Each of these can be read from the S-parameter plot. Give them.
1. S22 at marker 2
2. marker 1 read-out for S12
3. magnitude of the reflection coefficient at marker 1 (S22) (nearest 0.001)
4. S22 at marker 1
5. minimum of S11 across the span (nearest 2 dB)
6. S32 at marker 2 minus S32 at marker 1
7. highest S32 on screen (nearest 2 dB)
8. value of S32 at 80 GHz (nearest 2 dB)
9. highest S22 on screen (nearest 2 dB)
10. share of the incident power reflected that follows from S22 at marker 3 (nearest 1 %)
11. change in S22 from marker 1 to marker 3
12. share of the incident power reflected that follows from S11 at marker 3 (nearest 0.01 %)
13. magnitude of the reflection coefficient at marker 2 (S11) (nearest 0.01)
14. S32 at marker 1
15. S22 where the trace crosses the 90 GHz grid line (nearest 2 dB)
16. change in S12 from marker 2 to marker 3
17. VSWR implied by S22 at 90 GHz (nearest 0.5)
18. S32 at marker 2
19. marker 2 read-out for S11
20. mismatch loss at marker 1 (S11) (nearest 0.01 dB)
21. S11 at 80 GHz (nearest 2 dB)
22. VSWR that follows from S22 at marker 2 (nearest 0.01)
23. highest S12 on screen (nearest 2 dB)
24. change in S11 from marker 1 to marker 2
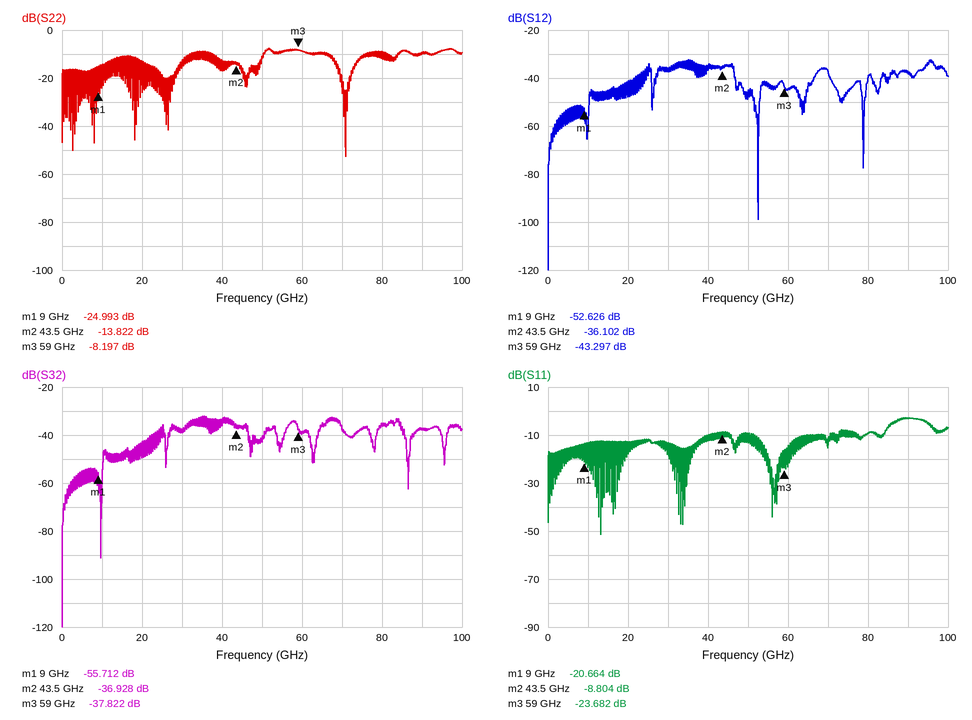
-13.822 dB
-52.626 dB
0.056
-24.993 dB
-52 dB
18.784 dB
-32 dB
-36 dB
-8 dB
15 %
16.796 dB
0.43 %
0.36
-55.712 dB
-10 dB
-7.195 dB
2.0
-36.928 dB
-8.804 dB
0.04 dB
-10 dB
1.51
-32 dB
11.860 dB
